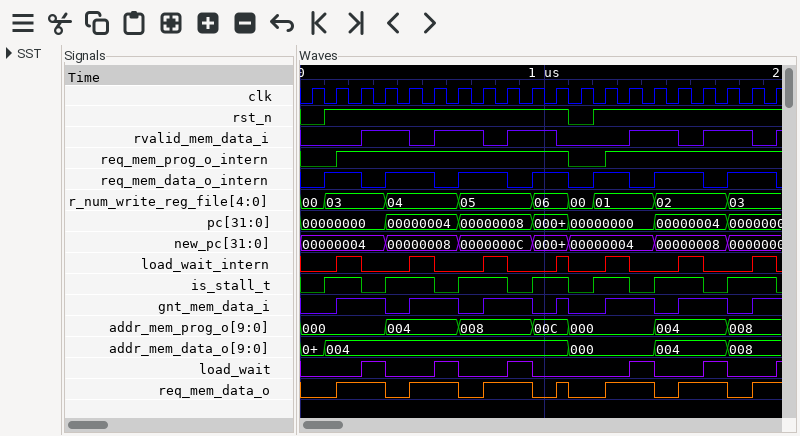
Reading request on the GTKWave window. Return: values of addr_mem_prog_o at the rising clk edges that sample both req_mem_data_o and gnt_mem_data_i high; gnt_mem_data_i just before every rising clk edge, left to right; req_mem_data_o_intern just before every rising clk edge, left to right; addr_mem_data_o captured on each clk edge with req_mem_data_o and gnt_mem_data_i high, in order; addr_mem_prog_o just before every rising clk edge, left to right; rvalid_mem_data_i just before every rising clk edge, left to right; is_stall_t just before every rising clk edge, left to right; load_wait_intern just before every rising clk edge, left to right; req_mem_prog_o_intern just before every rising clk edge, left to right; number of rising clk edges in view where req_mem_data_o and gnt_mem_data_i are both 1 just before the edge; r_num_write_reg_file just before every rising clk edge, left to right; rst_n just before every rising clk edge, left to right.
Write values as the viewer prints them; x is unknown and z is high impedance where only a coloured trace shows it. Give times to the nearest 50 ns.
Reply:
000, 000, 004, 004, 008, 008, 000, 000, 004, 004, 008
0 0 1 1 0 1 1 0 1 1 0 0 0 1 1 0 1 1 0 1
0 1 1 0 1 1 0 1 1 0 1 0 1 1 0 1 1 0 1 1
004, 004, 004, 004, 004, 004, 000, 000, 004, 004, 008
000, 000, 000, 000, 004, 004, 004, 008, 008, 008, 00C, 000, 000, 000, 000, 004, 004, 004, 008, 008
0 0 0 1 1 0 1 1 0 1 1 0 0 0 1 1 0 1 1 0
0 1 1 0 1 1 0 1 1 0 1 0 1 1 0 1 1 0 1 1
0 0 1 0 0 1 0 0 1 0 0 0 0 1 0 0 1 0 0 1
0 0 1 1 1 1 1 1 1 1 1 0 0 1 1 1 1 1 1 1
11
00, 03, 03, 03, 04, 04, 04, 05, 05, 05, 06, 00, 01, 01, 01, 02, 02, 02, 03, 03
0 1 1 1 1 1 1 1 1 1 1 0 1 1 1 1 1 1 1 1
